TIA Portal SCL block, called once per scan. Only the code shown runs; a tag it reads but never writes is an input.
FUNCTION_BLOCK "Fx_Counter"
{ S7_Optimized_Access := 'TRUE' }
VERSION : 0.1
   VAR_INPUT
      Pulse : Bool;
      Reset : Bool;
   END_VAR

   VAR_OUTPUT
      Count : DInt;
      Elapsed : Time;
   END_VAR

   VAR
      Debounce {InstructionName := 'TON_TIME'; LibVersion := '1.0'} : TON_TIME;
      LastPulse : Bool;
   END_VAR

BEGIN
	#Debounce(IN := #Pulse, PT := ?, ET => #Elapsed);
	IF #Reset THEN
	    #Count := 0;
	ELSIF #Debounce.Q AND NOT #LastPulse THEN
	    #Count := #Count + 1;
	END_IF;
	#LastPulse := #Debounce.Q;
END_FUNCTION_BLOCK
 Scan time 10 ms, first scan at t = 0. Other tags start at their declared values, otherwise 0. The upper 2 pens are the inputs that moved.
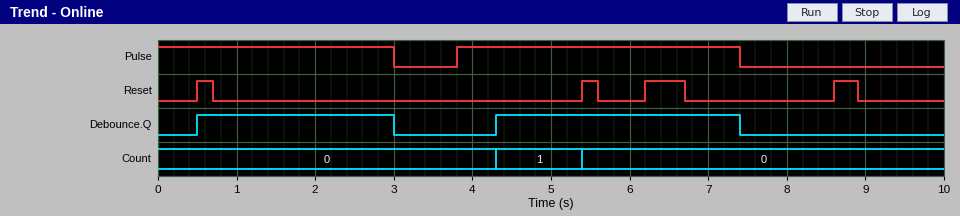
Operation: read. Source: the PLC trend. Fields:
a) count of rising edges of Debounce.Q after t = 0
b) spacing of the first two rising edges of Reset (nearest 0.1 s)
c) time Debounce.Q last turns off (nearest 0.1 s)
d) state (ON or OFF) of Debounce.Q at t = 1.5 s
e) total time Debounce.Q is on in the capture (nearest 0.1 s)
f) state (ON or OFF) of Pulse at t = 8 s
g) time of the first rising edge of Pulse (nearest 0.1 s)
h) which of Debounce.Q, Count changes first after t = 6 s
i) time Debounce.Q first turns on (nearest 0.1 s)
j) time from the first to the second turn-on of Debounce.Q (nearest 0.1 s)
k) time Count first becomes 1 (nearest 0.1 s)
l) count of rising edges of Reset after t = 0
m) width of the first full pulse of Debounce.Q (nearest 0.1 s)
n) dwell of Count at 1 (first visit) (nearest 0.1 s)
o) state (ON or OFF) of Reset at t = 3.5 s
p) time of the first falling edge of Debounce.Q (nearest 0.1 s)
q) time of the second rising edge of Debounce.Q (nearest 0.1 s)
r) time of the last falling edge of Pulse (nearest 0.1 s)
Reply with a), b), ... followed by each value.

a) 2
b) 4.9 s
c) 7.4 s
d) ON
e) 5.6 s
f) OFF
g) 3.8 s
h) Debounce.Q
i) 0.5 s
j) 3.8 s
k) 4.3 s
l) 4
m) 2.5 s
n) 1.1 s
o) OFF
p) 3.0 s
q) 4.3 s
r) 7.4 s
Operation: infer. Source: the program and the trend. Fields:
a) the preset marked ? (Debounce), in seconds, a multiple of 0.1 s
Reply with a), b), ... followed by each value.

a) 0.5 s
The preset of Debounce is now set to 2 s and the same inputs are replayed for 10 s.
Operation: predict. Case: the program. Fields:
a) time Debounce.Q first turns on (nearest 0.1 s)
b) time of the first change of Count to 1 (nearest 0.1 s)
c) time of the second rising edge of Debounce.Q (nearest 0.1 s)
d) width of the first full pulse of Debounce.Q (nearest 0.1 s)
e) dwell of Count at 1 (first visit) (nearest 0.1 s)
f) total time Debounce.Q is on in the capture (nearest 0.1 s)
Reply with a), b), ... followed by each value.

a) 2.0 s
b) 2.0 s
c) 5.8 s
d) 1.0 s
e) 3.4 s
f) 2.6 s
